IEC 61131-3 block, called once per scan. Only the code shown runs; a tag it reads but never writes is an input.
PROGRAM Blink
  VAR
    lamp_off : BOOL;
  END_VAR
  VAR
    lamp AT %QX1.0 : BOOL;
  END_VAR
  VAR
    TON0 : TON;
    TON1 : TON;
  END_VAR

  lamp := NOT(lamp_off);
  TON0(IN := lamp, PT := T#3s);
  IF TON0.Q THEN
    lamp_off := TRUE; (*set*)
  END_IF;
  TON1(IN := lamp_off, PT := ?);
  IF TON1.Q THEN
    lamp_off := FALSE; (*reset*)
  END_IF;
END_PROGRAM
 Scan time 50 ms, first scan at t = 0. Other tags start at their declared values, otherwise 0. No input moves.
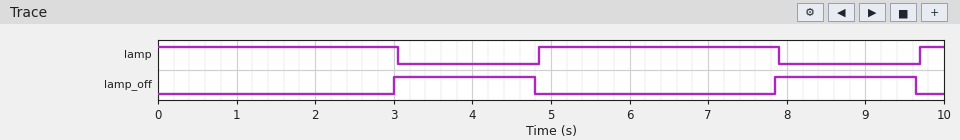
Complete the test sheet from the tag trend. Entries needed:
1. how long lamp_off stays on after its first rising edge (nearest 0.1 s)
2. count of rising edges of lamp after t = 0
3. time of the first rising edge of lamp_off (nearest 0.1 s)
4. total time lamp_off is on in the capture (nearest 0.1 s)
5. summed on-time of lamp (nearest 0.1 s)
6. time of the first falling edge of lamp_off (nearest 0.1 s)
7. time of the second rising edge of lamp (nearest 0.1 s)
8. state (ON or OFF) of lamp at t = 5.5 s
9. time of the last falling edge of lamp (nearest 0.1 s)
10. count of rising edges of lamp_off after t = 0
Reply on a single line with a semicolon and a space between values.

1.8 s; 2; 3.0 s; 3.6 s; 6.4 s; 4.8 s; 9.7 s; ON; 7.9 s; 2
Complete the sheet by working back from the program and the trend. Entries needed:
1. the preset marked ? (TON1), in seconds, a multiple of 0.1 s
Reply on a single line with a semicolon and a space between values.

1.8 s
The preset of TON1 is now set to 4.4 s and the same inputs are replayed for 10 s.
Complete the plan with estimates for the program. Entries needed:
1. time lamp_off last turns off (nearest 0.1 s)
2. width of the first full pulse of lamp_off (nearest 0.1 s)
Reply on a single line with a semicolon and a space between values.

7.4 s; 4.4 s
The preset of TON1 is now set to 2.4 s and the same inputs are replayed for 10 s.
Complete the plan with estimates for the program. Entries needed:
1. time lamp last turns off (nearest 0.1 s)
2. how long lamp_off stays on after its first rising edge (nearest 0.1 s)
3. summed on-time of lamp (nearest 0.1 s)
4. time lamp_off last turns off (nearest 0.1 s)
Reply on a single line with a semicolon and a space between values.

8.5 s; 2.4 s; 6.1 s; 5.4 s
